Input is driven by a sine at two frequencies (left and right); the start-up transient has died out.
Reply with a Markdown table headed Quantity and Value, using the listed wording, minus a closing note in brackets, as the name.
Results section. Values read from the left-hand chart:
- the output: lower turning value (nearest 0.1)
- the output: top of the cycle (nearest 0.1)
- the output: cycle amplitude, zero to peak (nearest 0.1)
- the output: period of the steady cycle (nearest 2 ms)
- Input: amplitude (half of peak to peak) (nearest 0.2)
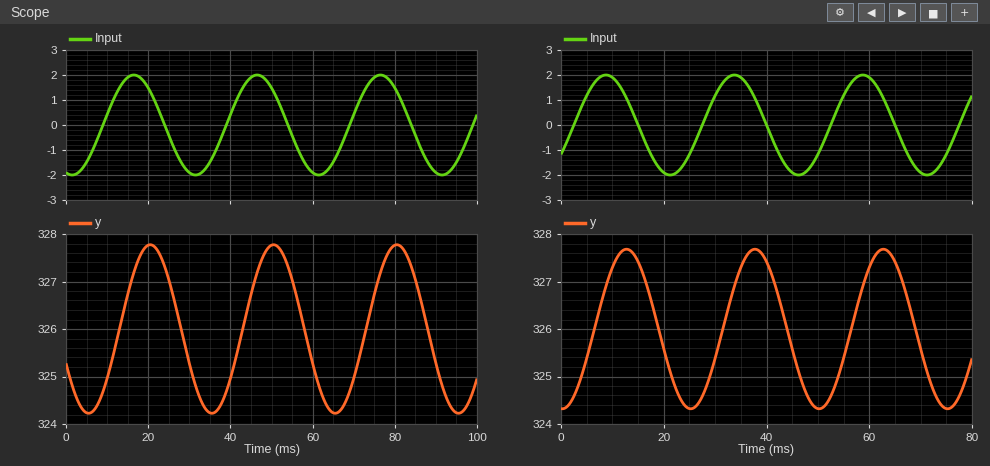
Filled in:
| Quantity | Value |
|---|---|
| the output: lower turning value | 324.2 |
| the output: top of the cycle | 327.8 |
| the output: cycle amplitude, zero to peak | 1.8 |
| the output: period of the steady cycle | 30 ms |
| Input: amplitude (half of peak to peak) | 2.0 |
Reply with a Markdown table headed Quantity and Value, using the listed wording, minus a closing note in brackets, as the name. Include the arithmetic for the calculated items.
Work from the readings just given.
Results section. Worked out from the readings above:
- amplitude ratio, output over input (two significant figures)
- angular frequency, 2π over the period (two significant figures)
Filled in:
| Quantity | Value |
|---|---|
| amplitude ratio, output over input | 1.8 / 2 = 0.90 |
| angular frequency, 2π over the period | 2π / 30 = 0.21 rad/ms |
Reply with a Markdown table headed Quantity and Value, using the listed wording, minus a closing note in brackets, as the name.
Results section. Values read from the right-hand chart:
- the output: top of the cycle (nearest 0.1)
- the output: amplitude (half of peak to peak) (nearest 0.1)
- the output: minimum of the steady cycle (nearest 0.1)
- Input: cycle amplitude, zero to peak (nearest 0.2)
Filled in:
| Quantity | Value |
|---|---|
| the output: top of the cycle | 327.7 |
| the output: amplitude (half of peak to peak) | 1.7 |
| the output: minimum of the steady cycle | 324.3 |
| Input: cycle amplitude, zero to peak | 2.0 |
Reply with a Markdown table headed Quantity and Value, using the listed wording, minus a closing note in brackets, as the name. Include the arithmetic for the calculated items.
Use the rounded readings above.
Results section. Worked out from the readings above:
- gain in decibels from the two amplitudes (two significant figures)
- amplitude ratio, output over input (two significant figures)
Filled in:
| Quantity | Value |
|---|---|
| gain in decibels from the two amplitudes | 20 log10(1.7 / 2) = -1.4 dB |
| amplitude ratio, output over input | 1.7 / 2 = 0.85 |
